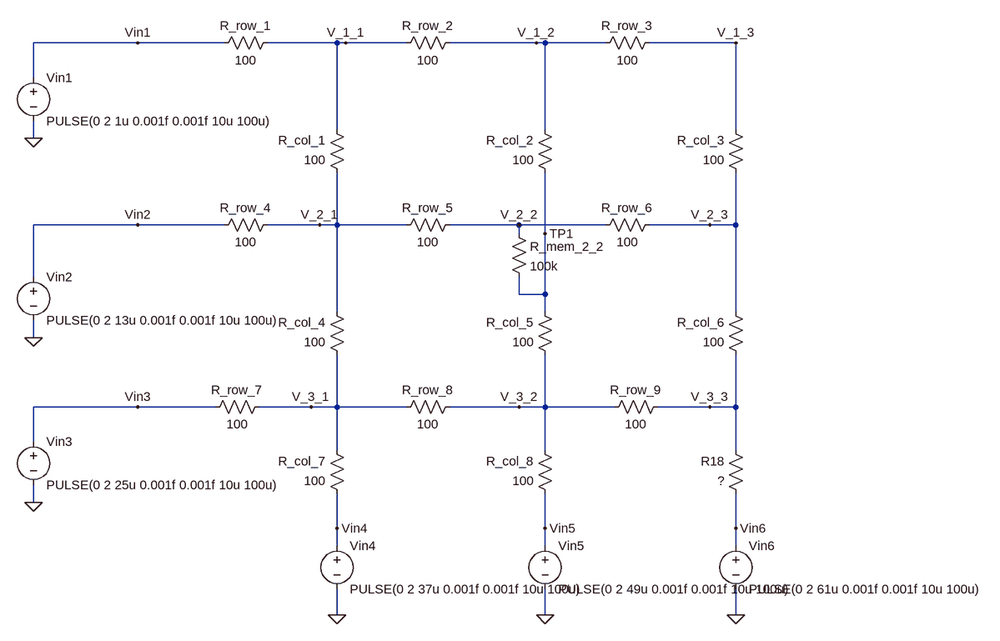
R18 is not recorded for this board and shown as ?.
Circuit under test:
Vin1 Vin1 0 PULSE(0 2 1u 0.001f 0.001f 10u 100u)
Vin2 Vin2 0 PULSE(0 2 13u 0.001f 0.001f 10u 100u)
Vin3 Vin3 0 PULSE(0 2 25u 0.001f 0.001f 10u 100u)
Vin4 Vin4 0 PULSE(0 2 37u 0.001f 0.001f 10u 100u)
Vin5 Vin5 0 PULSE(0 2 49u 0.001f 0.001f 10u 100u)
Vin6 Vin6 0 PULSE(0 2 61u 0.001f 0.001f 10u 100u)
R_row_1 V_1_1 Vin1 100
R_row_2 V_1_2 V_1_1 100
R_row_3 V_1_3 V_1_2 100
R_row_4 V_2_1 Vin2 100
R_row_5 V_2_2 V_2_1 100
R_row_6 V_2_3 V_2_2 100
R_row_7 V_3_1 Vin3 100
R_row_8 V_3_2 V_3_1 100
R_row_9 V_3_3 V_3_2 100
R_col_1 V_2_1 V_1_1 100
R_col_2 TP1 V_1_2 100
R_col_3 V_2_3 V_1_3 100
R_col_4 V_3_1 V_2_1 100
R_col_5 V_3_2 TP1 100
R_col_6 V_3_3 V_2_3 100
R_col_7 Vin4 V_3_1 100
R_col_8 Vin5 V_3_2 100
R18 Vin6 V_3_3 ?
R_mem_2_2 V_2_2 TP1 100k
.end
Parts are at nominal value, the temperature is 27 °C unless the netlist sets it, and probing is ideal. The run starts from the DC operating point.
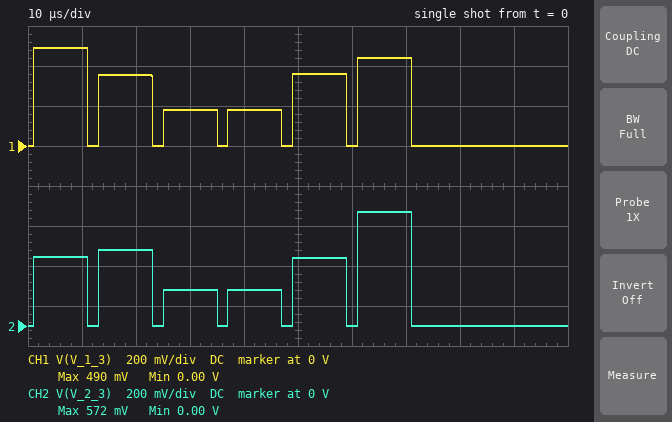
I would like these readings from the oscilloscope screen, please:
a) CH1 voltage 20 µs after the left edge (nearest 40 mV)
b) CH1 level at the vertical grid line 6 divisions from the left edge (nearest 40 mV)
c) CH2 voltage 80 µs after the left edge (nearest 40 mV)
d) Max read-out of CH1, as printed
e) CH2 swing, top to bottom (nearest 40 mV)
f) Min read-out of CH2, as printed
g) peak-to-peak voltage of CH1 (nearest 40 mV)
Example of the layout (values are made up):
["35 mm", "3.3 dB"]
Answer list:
["360 mV", "0 V", "0 V", "490 mV", "560 mV", "0.00 V", "480 mV"]
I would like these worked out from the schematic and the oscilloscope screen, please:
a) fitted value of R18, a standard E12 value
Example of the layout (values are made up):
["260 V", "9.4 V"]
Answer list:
["120 Ω"]
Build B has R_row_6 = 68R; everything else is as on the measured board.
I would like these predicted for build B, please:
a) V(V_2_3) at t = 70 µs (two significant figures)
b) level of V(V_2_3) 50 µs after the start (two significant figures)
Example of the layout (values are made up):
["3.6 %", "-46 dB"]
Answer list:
["550 mV", "330 mV"]
